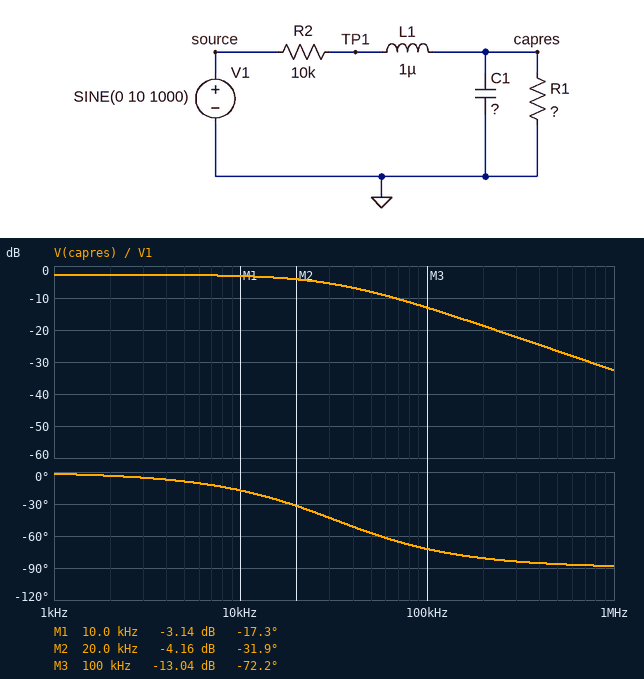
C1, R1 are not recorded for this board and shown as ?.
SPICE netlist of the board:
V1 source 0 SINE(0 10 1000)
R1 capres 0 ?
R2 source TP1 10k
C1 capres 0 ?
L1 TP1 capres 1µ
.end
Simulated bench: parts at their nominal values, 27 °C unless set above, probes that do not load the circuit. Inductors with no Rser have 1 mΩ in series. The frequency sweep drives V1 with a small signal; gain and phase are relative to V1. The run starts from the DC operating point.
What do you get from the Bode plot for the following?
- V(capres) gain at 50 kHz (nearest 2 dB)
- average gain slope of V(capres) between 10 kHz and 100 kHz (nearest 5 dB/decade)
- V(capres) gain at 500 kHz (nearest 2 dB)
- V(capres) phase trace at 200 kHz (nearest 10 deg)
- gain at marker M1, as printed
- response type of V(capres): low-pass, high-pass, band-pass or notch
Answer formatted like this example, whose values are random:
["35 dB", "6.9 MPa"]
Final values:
["-8 dB", "-10 dB/decade", "-26 dB", "-80 deg", "-3.14 dB", "low-pass"]
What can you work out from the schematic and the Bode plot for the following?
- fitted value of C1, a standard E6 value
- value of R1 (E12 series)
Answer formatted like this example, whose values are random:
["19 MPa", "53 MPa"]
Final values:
["680 pF", "27 kΩ"]
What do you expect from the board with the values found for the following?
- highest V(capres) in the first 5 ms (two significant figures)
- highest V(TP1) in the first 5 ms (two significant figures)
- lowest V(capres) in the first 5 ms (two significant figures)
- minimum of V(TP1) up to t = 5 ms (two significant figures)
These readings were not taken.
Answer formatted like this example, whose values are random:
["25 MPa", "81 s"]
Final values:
["7.3 V", "7.3 V", "-7.3 V", "-7.3 V"]
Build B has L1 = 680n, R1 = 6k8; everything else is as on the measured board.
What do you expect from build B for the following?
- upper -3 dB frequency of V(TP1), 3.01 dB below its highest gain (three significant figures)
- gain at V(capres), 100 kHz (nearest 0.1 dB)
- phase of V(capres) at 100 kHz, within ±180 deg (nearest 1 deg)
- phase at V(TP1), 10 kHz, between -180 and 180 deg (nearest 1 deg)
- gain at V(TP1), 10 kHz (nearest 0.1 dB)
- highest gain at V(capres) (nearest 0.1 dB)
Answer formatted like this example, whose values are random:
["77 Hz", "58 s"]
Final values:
["57.8 kHz", "-13.9 dB", "-60 deg", "-10 deg", "-8.0 dB", "-7.9 dB"]
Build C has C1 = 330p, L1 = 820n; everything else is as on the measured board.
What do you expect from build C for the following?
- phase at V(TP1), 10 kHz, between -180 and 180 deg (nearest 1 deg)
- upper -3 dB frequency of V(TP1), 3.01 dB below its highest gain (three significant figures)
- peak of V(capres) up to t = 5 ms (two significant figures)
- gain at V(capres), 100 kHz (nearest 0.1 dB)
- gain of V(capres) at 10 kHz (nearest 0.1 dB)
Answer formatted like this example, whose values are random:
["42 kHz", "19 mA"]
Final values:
["-9 deg", "66.1 kHz", "7.3 V", "-7.9 dB", "-2.8 dB"]
